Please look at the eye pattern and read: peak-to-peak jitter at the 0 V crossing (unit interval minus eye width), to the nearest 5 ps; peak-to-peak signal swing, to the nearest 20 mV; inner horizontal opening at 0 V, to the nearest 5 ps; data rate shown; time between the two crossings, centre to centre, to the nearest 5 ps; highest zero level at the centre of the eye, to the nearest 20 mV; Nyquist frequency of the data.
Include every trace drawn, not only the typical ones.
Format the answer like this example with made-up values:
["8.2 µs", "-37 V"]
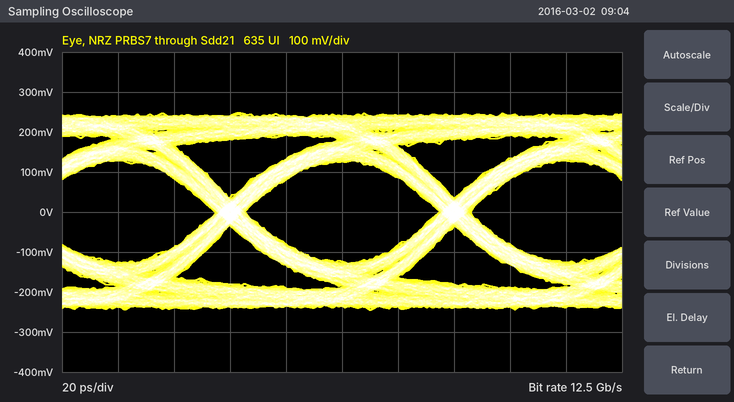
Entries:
["10 ps", "500 mV", "70 ps", "12.5 Gb/s", "80 ps", "-120 mV", "6.25 GHz"]
